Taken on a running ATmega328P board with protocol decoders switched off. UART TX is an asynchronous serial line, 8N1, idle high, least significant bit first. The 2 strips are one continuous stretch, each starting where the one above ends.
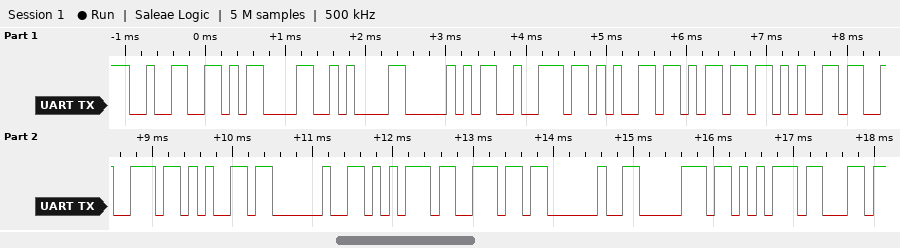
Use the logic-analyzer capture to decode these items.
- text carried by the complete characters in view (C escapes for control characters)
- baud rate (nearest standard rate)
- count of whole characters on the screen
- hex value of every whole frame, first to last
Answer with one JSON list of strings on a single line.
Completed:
["\"2\\r\\nPremere un pu\"", "9600 baud", "16", "0x32 0x0D 0x0A 0x50 0x72 0x65 0x6D 0x65 0x72 0x65 0x20 0x75 0x6E 0x20 0x70 0x75"]
